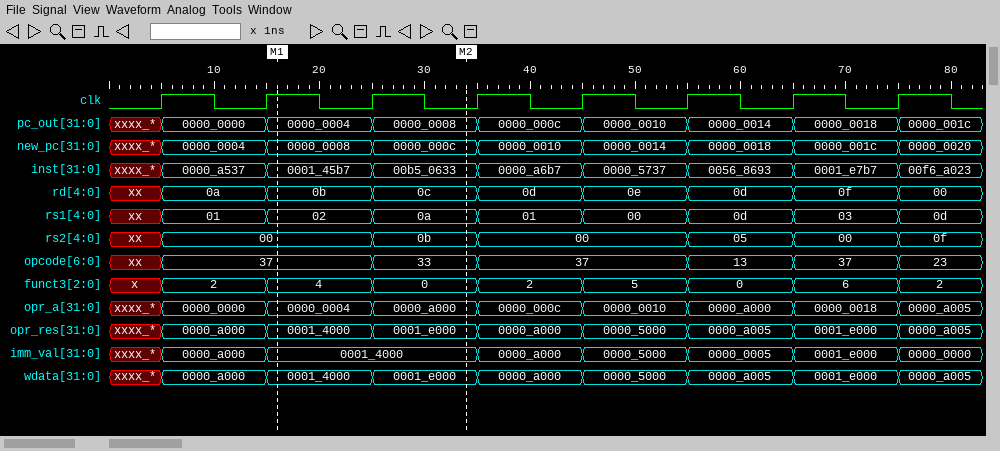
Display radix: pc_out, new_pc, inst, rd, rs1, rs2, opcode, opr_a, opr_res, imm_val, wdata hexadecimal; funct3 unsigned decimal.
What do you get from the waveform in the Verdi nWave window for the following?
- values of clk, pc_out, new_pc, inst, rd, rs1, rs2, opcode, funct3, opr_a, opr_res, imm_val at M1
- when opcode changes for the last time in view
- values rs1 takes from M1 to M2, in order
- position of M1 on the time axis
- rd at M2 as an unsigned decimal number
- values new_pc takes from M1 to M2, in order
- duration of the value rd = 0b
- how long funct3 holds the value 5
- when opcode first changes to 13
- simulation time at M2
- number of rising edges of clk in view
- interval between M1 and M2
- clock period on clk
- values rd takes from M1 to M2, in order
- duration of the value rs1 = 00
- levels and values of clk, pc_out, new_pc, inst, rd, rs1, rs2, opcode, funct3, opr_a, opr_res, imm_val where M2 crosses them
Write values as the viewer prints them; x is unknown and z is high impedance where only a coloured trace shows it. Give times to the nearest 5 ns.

clk=1, pc_out=0000_0004, new_pc=0000_0008, inst=0001_45b7, rd=0b, rs1=02, rs2=00, opcode=37, funct3=4, opr_a=0000_0004, opr_res=0001_4000, imm_val=0001_4000
75 ns
02, 0a
15 ns
12
0000_0008, 0000_000c
10 ns
10 ns
55 ns
35 ns
8
20 ns
10 ns
0b, 0c
10 ns
clk=0, pc_out=0000_0008, new_pc=0000_000c, inst=00b5_0633, rd=0c, rs1=0a, rs2=0b, opcode=33, funct3=0, opr_a=0000_a000, opr_res=0001_e000, imm_val=0001_4000
